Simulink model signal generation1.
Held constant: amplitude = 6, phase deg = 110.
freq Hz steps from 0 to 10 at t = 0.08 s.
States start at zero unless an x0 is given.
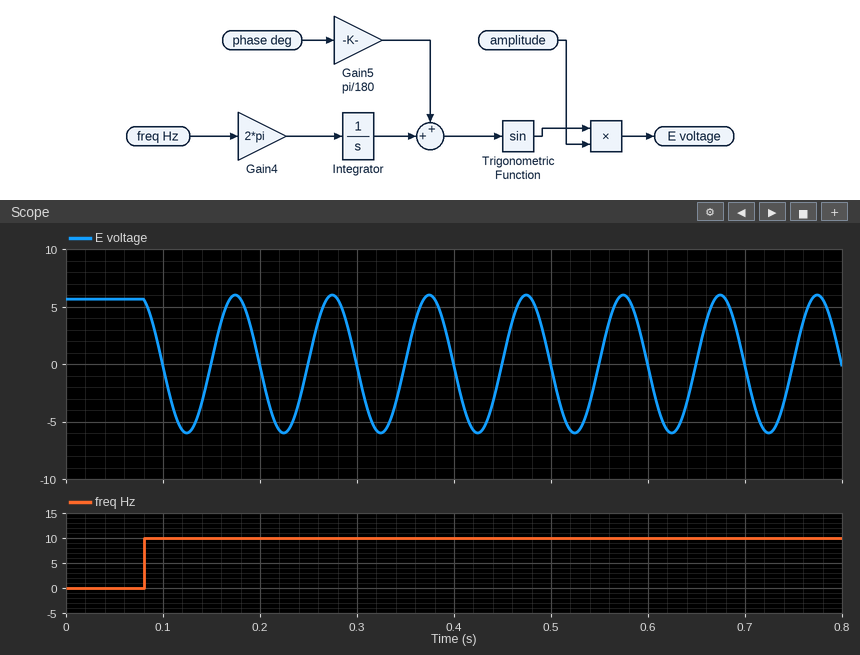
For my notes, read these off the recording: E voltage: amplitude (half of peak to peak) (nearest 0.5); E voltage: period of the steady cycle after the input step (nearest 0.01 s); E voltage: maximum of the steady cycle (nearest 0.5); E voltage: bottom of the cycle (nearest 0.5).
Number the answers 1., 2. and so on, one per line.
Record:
1. 6.0
2. 0.10 s
3. 6.0
4. -6.0
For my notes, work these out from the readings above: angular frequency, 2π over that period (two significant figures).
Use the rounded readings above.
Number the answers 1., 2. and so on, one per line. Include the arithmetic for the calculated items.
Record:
1. 2π / 0.1 = 63 rad/s
